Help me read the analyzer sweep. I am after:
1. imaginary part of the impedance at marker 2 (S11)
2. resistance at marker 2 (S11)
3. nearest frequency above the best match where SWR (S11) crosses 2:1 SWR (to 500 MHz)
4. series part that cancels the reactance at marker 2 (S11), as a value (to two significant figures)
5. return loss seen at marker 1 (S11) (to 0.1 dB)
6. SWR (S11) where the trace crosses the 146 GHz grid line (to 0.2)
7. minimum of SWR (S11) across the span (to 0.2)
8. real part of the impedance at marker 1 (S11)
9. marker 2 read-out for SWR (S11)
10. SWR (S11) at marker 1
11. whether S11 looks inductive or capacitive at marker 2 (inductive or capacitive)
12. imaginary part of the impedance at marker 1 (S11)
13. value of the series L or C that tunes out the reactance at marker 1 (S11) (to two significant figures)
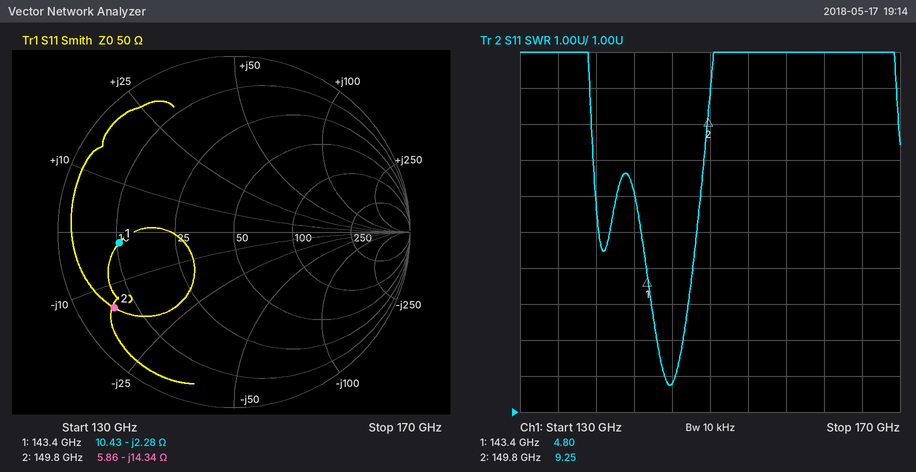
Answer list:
-14.34 Ω
5.86 Ω
146.5 GHz
15 pH
3.7 dB
1.8
1.8
10.43 Ω
9.25
4.80
capacitive
-2.28 Ω
2.5 pH
